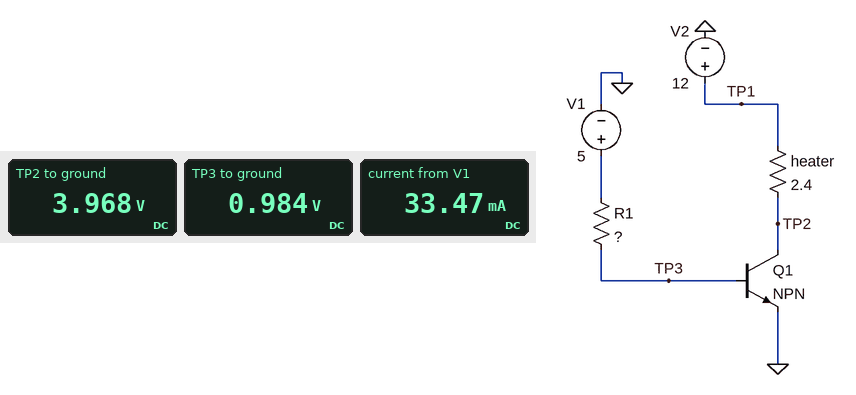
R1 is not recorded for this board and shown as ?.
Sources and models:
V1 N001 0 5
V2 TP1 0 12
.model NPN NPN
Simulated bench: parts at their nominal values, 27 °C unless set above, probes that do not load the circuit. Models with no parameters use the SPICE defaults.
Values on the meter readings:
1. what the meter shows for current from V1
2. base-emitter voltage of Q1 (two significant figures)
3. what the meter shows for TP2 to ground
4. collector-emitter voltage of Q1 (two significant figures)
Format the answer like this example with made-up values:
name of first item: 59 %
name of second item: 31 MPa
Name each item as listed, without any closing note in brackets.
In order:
what the meter shows for current from V1: 33.47 mA
base-emitter voltage of Q1: 980 mV
what the meter shows for TP2 to ground: 3.968 V
collector-emitter voltage of Q1: 4.0 V
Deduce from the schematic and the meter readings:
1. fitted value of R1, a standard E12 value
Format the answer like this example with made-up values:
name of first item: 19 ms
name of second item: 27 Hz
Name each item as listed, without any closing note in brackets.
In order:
fitted value of R1, a standard E12 value: 120 Ω
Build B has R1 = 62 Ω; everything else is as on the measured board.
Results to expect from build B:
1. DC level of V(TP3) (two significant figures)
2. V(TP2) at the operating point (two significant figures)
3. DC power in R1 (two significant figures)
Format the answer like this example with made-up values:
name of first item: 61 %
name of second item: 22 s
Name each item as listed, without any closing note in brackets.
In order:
DC level of V(TP3): 990 mV
V(TP2) at the operating point: 150 mV
DC power in R1: 260 mW
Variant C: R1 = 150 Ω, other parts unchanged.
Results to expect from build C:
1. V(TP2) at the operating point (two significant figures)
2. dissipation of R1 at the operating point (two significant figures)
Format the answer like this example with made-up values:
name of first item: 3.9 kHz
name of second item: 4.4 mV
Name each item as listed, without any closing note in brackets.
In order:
V(TP2) at the operating point: 5.6 V
dissipation of R1 at the operating point: 110 mW
